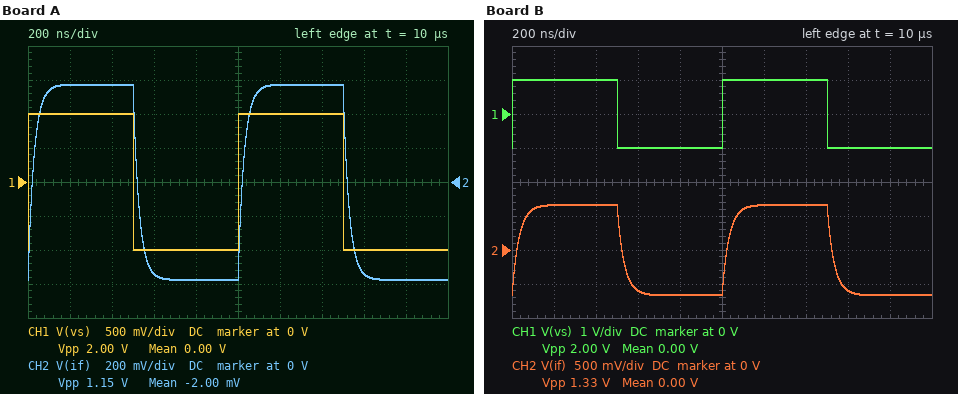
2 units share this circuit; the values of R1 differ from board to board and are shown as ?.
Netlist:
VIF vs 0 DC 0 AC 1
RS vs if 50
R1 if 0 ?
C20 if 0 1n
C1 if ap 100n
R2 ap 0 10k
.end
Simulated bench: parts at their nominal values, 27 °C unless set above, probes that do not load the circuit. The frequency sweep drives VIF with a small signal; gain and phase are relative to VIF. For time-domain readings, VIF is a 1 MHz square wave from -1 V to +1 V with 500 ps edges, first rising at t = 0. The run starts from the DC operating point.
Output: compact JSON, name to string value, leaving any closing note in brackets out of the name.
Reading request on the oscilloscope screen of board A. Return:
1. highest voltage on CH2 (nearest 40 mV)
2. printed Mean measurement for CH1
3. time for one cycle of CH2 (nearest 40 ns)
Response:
{"highest voltage on CH2": "560 mV", "printed Mean measurement for CH1": "0.00 V", "time for one cycle of CH2": "1.00 µs"}
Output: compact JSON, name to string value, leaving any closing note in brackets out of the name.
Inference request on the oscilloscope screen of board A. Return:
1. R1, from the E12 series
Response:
{"R1, from the E12 series": "68 Ω"}
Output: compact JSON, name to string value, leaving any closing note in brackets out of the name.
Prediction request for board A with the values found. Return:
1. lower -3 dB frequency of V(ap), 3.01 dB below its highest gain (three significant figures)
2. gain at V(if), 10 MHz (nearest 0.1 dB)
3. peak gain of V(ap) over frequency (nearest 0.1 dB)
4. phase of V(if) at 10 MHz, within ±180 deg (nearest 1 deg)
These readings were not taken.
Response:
{"lower -3 dB frequency of V(ap), 3.01 dB below its highest gain": "159 Hz", "gain at V(if), 10 MHz": "-11.1 dB", "peak gain of V(ap) over frequency": "-4.8 dB", "phase of V(if) at 10 MHz, within ±180 deg": "-61 deg"}
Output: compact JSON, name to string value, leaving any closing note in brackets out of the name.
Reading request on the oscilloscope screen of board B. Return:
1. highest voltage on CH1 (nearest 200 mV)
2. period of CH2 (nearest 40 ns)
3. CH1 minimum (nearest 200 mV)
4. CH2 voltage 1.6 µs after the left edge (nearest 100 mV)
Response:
{"highest voltage on CH1": "1.0 V", "period of CH2": "1.00 µs", "CH1 minimum": "-1.0 V", "CH2 voltage 1.6 µs after the left edge": "-600 mV"}
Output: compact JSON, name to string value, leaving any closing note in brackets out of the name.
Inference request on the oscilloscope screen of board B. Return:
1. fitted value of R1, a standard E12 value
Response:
{"fitted value of R1, a standard E12 value": "100 Ω"}
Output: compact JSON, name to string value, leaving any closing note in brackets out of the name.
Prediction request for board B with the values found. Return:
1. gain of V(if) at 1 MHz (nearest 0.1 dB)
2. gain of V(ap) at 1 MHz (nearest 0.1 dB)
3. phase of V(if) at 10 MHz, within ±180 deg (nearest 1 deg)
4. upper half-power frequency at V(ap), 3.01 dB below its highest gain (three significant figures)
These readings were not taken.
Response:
{"gain of V(if) at 1 MHz": "-3.7 dB", "gain of V(ap) at 1 MHz": "-3.7 dB", "phase of V(if) at 10 MHz, within ±180 deg": "-64 deg", "upper half-power frequency at V(ap), 3.01 dB below its highest gain": "4.79 MHz"}
